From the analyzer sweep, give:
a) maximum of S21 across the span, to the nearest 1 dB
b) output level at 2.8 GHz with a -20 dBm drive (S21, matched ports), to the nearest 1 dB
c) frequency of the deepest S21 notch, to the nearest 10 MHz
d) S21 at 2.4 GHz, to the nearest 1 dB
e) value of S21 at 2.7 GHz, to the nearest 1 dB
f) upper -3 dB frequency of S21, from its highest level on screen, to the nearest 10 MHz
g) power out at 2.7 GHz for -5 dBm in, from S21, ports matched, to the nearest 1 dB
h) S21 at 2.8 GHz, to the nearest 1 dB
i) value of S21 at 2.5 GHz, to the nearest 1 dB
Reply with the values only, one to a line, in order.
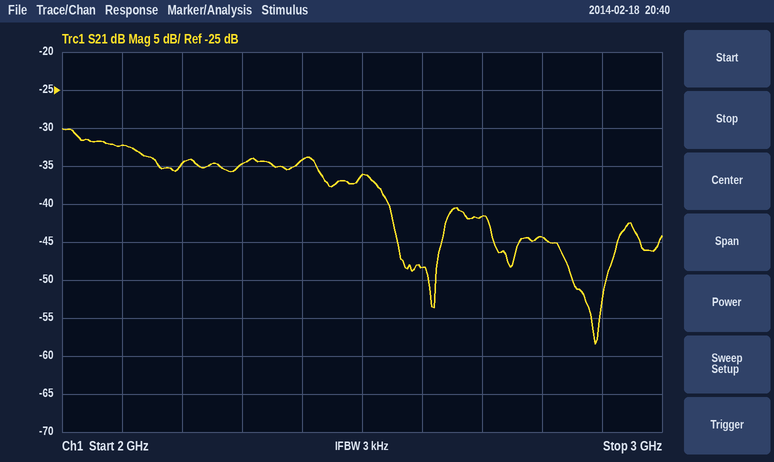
-30 dB
-64 dBm
2.89 GHz
-34 dB
-42 dB
2.13 GHz
-47 dBm
-44 dB
-36 dB
